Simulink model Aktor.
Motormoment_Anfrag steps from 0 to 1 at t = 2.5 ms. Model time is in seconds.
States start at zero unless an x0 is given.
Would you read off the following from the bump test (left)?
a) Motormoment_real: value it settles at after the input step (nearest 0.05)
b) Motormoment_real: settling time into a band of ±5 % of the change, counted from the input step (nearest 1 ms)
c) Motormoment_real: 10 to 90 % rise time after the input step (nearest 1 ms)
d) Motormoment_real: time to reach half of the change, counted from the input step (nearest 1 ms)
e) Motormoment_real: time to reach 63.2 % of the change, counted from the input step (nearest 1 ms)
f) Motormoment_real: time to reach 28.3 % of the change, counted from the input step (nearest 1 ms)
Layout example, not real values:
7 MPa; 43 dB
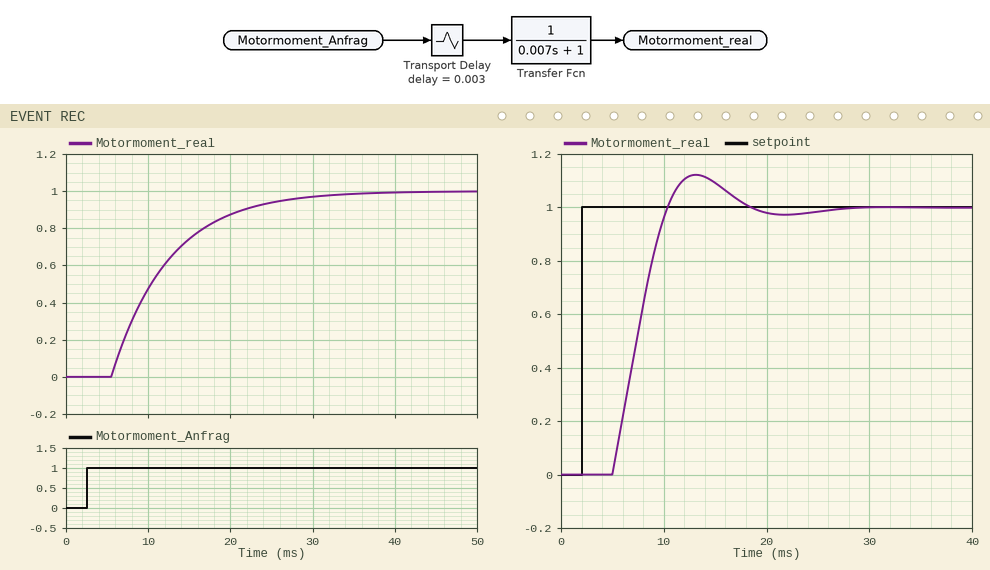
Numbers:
1.00; 24 ms; 15 ms; 8 ms; 10 ms; 5 ms
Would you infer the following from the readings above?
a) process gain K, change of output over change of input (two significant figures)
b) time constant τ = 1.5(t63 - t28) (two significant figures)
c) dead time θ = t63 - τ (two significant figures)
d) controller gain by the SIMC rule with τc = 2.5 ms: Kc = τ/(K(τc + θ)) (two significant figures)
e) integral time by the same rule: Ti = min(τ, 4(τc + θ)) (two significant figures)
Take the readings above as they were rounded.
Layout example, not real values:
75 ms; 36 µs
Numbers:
1.0; 7.5 ms; 2.5 ms; 1.5; 7.5 ms
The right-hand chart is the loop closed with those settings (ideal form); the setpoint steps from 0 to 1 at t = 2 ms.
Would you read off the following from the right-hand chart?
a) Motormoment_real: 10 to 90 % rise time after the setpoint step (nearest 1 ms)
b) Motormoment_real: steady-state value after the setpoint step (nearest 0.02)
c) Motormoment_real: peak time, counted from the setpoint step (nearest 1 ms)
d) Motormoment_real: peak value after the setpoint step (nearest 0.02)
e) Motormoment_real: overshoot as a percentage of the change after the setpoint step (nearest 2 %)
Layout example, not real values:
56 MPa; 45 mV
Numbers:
4 ms; 1.00; 11 ms; 1.12; 12 %
